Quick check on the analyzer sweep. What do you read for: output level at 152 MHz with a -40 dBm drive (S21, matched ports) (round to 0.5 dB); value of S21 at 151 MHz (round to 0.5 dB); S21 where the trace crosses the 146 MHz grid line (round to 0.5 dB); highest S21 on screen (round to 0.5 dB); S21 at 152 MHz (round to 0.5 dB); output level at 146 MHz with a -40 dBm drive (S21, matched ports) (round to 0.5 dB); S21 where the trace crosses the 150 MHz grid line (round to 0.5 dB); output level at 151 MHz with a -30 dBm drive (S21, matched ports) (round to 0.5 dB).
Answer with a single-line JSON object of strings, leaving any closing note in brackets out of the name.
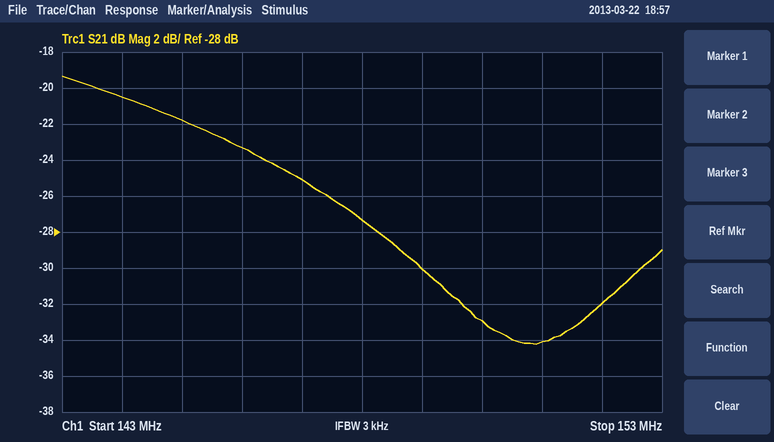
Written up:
{"output level at 152 MHz with a -40 dBm drive (S21, matched ports)": "-72.0 dBm", "value of S21 at 151 MHz": "-34.0 dB", "S21 where the trace crosses the 146 MHz grid line": "-23.5 dB", "highest S21 on screen": "-19.5 dB", "S21 at 152 MHz": "-32.0 dB", "output level at 146 MHz with a -40 dBm drive (S21, matched ports)": "-63.5 dBm", "S21 where the trace crosses the 150 MHz grid line": "-33.0 dB", "output level at 151 MHz with a -30 dBm drive (S21, matched ports)": "-64.0 dBm"}
